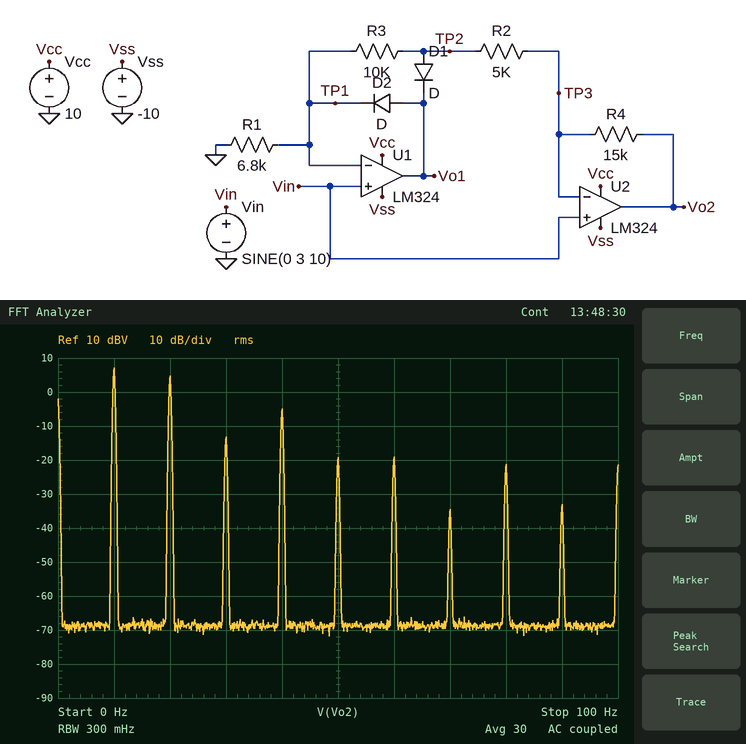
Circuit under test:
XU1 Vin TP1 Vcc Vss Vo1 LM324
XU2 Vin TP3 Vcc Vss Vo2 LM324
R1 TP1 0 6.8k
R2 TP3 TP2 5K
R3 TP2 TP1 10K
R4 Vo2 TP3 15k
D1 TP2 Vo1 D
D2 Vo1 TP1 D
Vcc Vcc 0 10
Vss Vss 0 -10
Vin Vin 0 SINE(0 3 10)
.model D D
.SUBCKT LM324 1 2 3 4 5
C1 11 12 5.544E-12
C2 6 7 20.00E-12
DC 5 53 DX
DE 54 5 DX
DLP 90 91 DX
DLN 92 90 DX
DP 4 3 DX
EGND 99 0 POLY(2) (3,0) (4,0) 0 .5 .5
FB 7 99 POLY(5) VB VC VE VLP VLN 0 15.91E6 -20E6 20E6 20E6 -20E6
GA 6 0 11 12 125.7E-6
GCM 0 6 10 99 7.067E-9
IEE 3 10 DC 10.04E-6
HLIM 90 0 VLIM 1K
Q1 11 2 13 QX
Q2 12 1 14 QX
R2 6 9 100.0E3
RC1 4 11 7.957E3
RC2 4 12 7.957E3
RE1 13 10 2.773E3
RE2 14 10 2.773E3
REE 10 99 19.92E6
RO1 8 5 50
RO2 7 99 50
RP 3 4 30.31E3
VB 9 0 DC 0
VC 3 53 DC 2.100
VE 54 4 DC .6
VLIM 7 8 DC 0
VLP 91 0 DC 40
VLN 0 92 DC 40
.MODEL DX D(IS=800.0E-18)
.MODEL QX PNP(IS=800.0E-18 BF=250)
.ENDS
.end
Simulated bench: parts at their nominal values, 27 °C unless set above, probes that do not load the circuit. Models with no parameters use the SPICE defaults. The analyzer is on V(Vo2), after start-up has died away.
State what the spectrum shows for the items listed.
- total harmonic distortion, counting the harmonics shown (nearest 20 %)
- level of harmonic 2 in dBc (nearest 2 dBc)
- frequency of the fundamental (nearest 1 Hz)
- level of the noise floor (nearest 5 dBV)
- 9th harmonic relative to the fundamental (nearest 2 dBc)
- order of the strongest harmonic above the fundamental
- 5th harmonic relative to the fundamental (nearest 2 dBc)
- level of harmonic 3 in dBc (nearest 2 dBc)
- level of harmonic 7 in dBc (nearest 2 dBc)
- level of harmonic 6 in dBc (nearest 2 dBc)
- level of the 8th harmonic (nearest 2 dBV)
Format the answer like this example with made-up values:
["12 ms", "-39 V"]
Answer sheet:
["80 %", "-2 dBc", "10 Hz", "-70 dBV", "-40 dBc", "2", "-26 dBc", "-20 dBc", "-42 dBc", "-26 dBc", "-22 dBV"]
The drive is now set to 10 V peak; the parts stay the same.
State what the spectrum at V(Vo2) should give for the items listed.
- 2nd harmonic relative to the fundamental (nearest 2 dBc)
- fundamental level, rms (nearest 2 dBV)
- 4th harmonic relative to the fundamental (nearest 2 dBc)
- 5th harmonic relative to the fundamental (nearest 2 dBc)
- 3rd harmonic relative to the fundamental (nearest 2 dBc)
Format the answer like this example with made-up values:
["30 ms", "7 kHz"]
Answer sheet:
["-8 dBc", "14 dBV", "-14 dBc", "-12 dBc", "-6 dBc"]
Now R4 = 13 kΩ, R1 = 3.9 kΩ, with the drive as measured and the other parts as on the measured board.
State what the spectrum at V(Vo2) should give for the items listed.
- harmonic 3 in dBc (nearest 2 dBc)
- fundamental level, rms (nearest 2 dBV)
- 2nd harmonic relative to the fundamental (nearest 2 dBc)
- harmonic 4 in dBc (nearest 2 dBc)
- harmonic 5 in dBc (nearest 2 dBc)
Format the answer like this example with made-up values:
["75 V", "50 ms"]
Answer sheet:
["-10 dBc", "8 dBV", "-6 dBc", "-10 dBc", "-24 dBc"]
